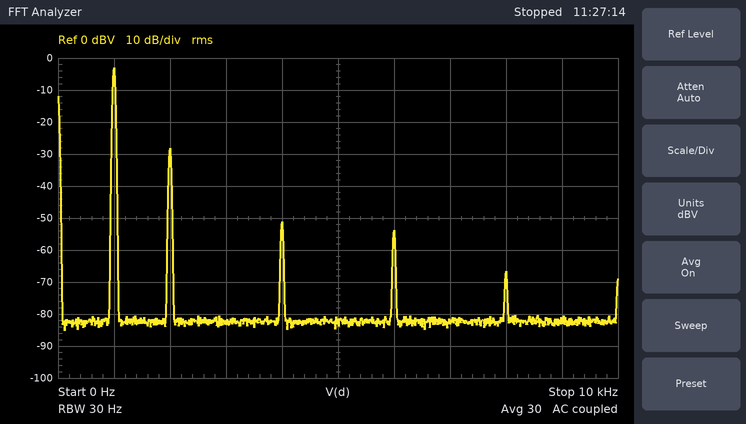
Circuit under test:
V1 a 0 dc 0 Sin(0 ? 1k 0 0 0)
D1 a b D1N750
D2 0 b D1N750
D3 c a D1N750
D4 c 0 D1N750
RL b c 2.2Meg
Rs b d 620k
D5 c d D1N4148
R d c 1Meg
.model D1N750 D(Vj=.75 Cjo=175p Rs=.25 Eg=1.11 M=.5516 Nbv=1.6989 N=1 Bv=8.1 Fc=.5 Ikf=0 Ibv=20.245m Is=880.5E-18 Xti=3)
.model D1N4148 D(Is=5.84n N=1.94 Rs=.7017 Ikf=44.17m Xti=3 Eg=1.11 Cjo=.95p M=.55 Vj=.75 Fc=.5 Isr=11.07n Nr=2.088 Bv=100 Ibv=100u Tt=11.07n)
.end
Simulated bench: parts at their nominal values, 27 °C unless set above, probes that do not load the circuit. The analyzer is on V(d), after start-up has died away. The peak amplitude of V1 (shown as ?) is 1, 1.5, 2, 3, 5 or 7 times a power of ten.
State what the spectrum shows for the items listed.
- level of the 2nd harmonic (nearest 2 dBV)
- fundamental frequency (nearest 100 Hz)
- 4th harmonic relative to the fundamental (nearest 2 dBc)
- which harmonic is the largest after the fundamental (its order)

-28 dBV
1.0 kHz
-48 dBc
2
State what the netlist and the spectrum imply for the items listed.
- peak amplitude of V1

2 V
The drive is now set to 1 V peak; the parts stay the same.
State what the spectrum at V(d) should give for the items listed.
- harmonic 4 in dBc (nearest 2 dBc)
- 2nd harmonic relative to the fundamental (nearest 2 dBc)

-54 dBc
-42 dBc
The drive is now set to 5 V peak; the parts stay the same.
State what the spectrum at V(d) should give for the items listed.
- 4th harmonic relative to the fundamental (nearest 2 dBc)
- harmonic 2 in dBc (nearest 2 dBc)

-42 dBc
-22 dBc
